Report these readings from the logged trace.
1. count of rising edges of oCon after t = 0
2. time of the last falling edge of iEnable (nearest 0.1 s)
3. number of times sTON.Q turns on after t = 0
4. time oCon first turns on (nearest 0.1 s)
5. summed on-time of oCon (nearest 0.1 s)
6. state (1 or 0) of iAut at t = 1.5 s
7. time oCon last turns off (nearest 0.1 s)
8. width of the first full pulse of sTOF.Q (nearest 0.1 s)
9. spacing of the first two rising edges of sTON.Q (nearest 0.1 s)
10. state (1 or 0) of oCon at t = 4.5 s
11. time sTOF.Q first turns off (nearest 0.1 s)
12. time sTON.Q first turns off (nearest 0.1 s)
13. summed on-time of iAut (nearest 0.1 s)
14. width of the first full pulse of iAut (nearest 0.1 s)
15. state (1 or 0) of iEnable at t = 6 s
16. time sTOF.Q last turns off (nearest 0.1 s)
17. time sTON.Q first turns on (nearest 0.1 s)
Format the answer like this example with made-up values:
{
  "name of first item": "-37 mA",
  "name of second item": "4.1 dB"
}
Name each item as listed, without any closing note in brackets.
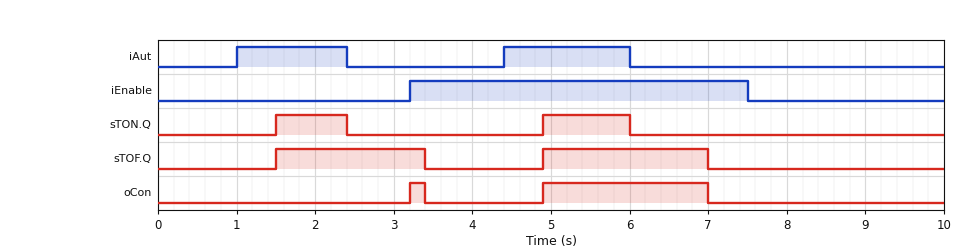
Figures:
{
  "count of rising edges of oCon after t = 0": "2",
  "time of the last falling edge of iEnable": "7.5 s",
  "number of times sTON.Q turns on after t = 0": "2",
  "time oCon first turns on": "3.2 s",
  "summed on-time of oCon": "2.3 s",
  "state (1 or 0) of iAut at t = 1.5 s": "1",
  "time oCon last turns off": "7.0 s",
  "width of the first full pulse of sTOF.Q": "1.9 s",
  "spacing of the first two rising edges of sTON.Q": "3.4 s",
  "state (1 or 0) of oCon at t = 4.5 s": "0",
  "time sTOF.Q first turns off": "3.4 s",
  "time sTON.Q first turns off": "2.4 s",
  "summed on-time of iAut": "3.0 s",
  "width of the first full pulse of iAut": "1.4 s",
  "state (1 or 0) of iEnable at t = 6 s": "1",
  "time sTOF.Q last turns off": "7.0 s",
  "time sTON.Q first turns on": "1.5 s"
}
